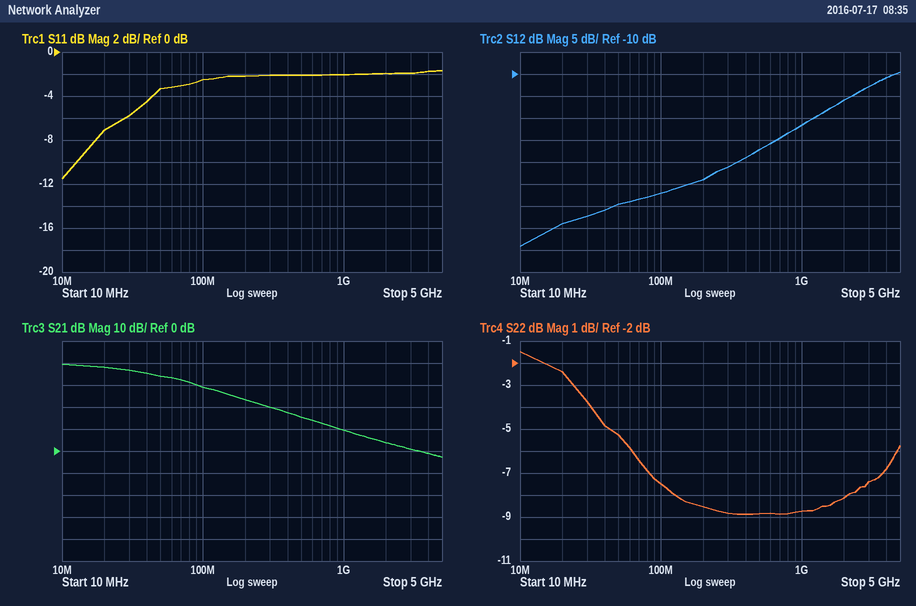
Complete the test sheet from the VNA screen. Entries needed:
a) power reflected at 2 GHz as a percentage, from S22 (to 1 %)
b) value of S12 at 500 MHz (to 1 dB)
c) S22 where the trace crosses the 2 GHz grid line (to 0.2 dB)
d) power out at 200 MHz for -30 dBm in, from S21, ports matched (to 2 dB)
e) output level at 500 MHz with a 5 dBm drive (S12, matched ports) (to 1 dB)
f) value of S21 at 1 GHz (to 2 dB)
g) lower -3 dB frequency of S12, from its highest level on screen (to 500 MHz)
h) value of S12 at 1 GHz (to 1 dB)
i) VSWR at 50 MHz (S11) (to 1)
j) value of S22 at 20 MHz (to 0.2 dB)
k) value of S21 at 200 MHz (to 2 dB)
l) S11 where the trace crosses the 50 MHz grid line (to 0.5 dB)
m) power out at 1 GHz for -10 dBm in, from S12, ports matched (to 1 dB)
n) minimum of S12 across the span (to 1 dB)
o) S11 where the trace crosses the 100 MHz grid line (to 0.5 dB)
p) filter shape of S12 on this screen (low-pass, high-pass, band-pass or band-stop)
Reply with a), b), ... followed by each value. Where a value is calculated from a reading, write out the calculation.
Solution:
a) 10^(-8.2/10) ≈ 15 %
b) -27 dB
c) -8.2 dB
d) -30 dBm + (24 dB) = -6 dBm
e) 5 dBm + (-27 dB) = -22 dBm
f) 10 dB
g) 3.0 GHz
h) -22 dB
i) |Γ| = 10^(-3.5/20) = 0.6683; VSWR = (1 + 0.6683)/(1 − 0.6683) ≈ 5
j) -2.4 dB
k) 24 dB
l) -3.5 dB
m) -10 dBm + (-22 dB) = -32 dBm
n) -49 dB
o) -2.5 dB
p) high-pass
